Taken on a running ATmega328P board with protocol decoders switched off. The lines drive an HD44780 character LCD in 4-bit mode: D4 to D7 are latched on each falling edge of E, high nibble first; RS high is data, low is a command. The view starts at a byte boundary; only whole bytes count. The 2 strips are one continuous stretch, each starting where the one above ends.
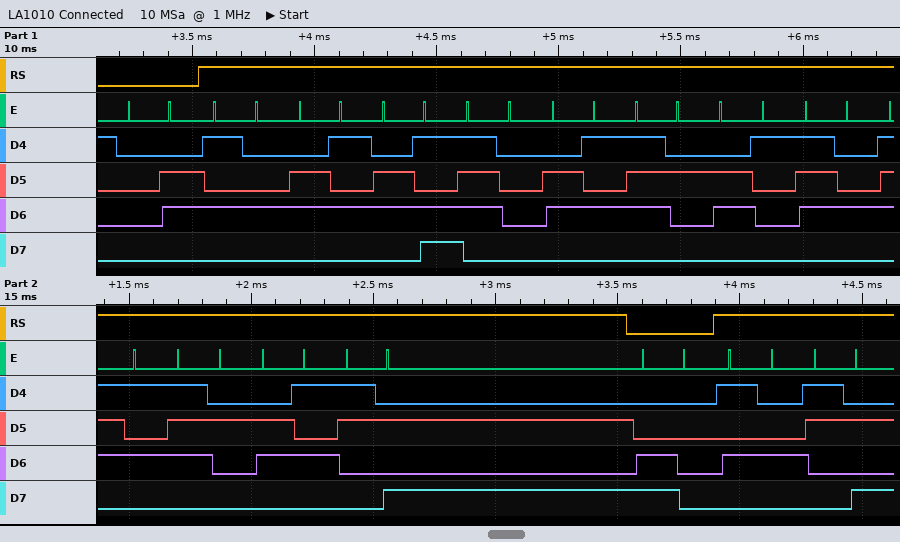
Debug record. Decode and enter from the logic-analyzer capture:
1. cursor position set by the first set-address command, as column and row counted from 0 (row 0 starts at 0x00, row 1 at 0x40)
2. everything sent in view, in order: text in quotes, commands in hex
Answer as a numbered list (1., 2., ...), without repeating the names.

1. column 0, row 1
2. 0x06 "Temperature:" 0xC0 "T:"
